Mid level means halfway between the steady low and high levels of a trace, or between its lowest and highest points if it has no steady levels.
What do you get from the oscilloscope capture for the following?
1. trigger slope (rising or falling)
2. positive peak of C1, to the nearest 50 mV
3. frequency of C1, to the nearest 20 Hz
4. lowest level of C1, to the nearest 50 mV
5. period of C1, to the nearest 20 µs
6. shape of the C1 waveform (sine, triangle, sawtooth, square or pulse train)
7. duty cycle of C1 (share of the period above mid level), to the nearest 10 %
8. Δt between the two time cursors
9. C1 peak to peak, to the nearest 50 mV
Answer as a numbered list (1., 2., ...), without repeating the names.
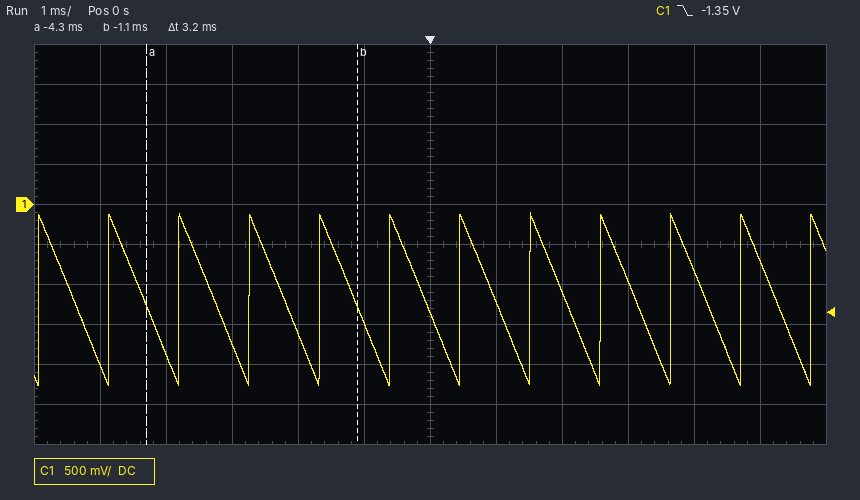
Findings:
1. falling
2. -100 mV
3. 940 Hz
4. -2.25 V
5. 1.06 ms
6. sawtooth
7. 50 %
8. 3.2 ms
9. 2.15 V
